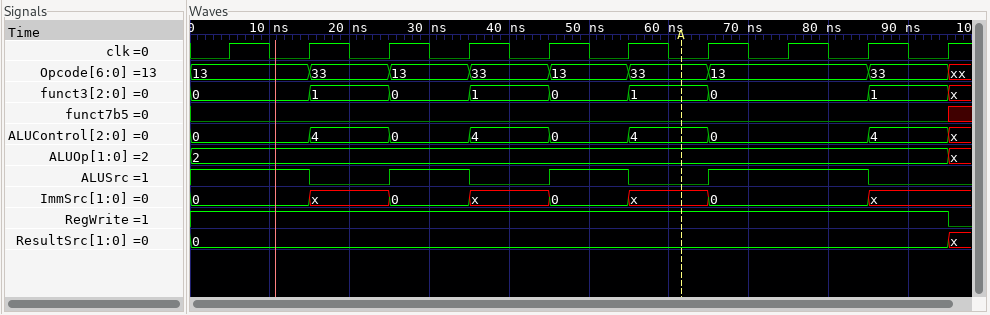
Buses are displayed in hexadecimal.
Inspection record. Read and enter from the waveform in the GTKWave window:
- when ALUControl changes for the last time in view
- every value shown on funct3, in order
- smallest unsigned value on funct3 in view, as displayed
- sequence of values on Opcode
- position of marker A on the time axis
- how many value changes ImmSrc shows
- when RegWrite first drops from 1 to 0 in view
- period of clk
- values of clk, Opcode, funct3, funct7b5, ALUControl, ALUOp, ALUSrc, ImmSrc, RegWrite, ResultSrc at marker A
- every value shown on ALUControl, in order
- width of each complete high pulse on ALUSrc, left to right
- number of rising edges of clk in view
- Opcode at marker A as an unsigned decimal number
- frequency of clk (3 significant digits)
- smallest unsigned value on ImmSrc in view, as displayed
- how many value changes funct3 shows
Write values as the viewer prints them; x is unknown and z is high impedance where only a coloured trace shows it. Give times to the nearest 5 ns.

95 ns
0, 1, 0, 1, 0, 1, 0, 1, x
0
13, 33, 13, 33, 13, 33, 13, 33, xx
60 ns
7
95 ns
10 ns
clk=0, Opcode=33, funct3=1, funct7b5=0, ALUControl=4, ALUOp=2, ALUSrc=0, ImmSrc=x, RegWrite=1, ResultSrc=0
0, 4, 0, 4, 0, 4, 0, 4, x
10 ns, 10 ns, 20 ns
10
51
100 MHz
0
8
